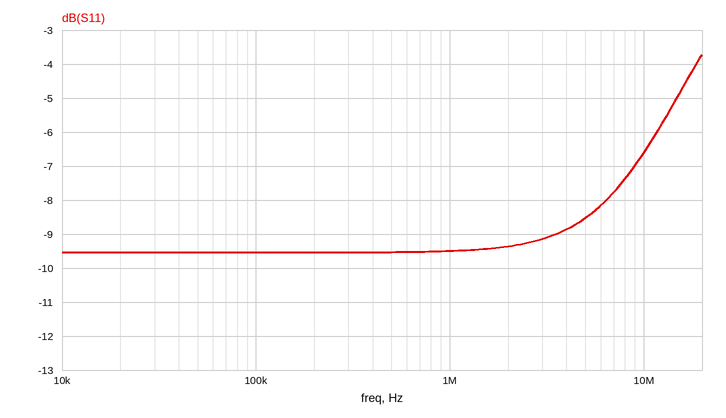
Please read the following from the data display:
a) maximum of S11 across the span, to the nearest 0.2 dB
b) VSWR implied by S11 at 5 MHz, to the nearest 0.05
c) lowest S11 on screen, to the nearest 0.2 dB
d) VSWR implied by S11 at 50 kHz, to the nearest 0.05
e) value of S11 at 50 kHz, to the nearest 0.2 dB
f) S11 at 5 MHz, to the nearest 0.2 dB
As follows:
-3.8 dB
2.20
-9.6 dB
2.00
-9.6 dB
-8.6 dB
